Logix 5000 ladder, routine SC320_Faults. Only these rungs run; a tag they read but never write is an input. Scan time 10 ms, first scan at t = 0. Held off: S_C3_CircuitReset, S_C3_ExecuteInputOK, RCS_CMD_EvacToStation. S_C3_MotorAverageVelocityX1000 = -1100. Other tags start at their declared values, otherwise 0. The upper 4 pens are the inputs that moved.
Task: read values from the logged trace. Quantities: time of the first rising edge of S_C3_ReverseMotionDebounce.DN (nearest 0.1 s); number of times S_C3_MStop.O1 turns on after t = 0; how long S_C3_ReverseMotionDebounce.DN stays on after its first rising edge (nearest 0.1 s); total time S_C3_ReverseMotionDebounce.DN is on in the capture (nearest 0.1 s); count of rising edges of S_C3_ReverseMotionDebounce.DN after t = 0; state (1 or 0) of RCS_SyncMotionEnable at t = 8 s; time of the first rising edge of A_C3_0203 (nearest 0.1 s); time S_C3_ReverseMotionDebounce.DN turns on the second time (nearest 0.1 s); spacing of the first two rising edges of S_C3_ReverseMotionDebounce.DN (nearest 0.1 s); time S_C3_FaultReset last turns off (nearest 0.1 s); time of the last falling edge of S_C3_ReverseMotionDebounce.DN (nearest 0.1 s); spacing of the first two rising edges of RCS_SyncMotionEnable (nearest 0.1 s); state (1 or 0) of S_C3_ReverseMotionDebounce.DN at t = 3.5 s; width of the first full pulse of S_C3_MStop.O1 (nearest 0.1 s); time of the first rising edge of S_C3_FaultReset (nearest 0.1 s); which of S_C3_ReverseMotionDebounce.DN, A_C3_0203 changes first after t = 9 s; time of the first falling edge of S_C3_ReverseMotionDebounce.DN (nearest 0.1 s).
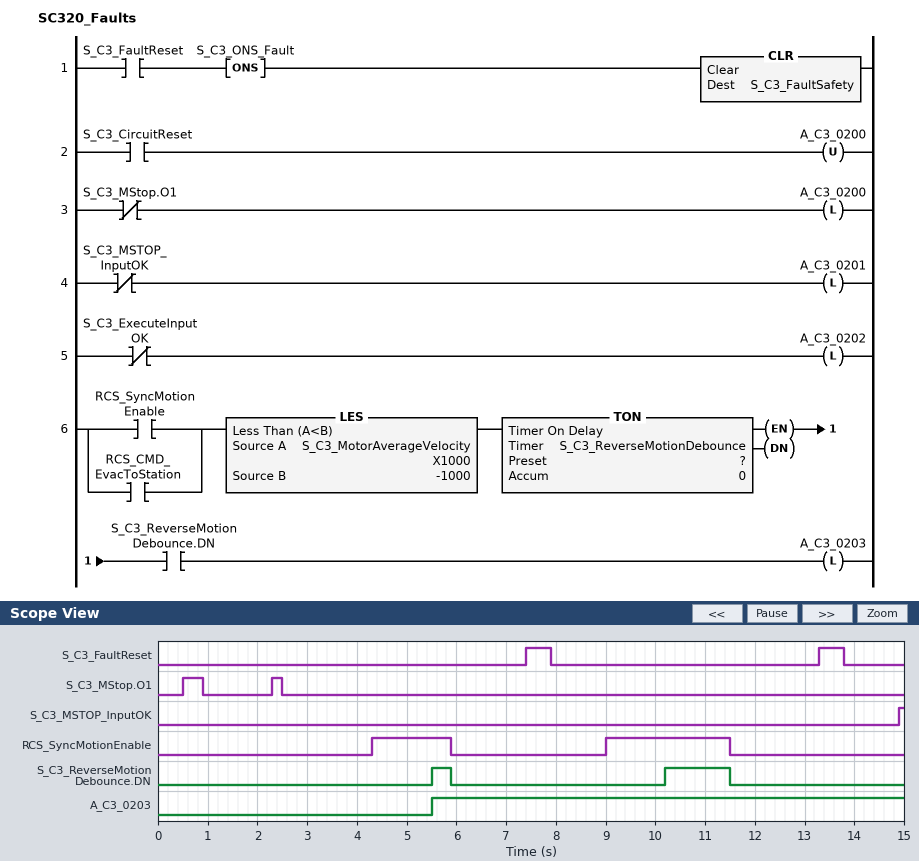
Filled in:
5.5 s
2
0.4 s
1.7 s
2
0
5.5 s
10.2 s
4.7 s
13.8 s
11.5 s
4.7 s
0
0.4 s
7.4 s
S_C3_ReverseMotionDebounce.DN
5.9 s
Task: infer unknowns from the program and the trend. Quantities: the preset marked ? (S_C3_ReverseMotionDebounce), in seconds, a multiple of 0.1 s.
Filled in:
1.2 s
